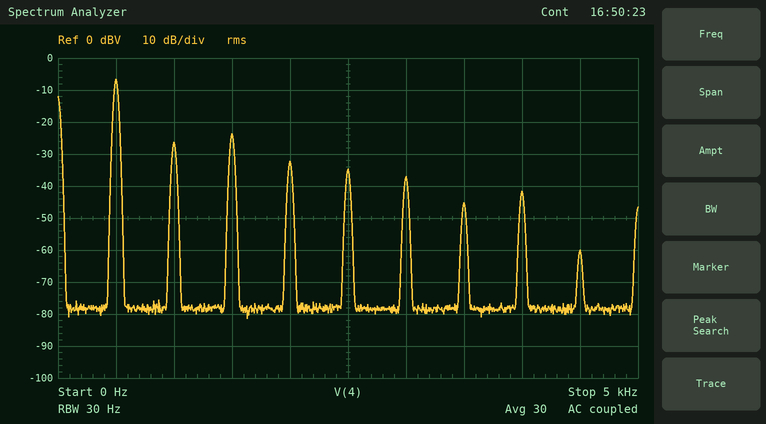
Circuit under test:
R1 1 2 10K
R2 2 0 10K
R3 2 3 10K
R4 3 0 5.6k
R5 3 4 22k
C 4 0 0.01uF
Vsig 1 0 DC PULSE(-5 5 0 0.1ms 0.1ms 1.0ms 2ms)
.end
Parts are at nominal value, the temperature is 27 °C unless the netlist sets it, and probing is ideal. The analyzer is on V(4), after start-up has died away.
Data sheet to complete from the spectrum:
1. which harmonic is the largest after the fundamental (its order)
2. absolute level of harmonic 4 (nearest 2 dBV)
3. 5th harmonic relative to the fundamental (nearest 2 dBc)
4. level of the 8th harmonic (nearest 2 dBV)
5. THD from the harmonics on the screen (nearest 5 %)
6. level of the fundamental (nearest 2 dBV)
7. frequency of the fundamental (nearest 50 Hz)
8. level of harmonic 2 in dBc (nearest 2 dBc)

3
-32 dBV
-28 dBc
-42 dBV
20 %
-6 dBV
500 Hz
-20 dBc
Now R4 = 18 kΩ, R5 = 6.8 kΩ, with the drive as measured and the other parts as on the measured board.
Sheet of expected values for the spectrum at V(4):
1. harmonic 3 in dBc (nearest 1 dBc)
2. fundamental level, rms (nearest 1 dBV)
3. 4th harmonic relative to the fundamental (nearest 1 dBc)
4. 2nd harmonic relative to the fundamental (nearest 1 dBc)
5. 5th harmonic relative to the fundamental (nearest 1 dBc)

-15 dBc
1 dBV
-23 dBc
-18 dBc
-25 dBc
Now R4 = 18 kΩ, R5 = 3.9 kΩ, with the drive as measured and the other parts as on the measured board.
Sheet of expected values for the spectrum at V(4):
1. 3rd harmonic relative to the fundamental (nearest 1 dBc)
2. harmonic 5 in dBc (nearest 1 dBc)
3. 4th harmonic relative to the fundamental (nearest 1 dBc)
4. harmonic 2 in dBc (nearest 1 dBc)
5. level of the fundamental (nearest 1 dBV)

-14 dBc
-24 dBc
-22 dBc
-18 dBc
1 dBV
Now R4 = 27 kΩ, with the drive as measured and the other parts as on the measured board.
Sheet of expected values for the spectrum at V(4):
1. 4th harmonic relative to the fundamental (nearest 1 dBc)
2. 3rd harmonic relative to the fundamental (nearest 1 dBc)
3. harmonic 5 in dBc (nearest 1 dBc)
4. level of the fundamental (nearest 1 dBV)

-26 dBc
-18 dBc
-29 dBc
0 dBV
